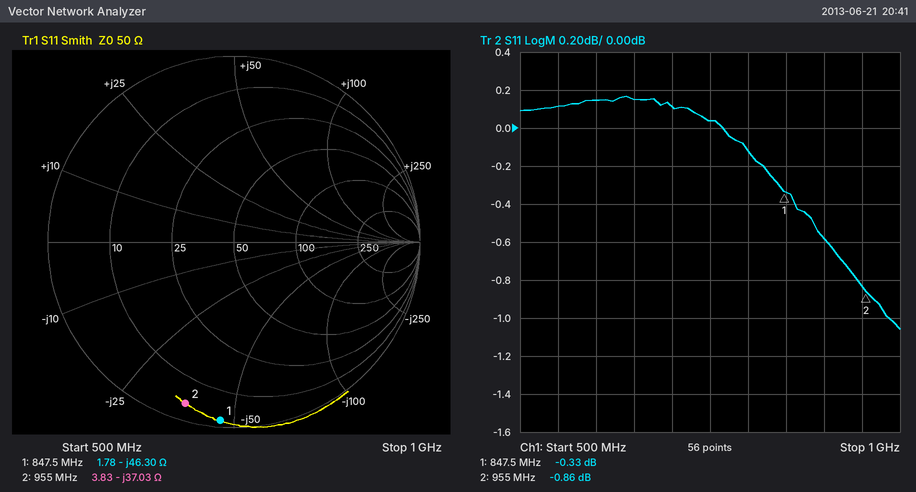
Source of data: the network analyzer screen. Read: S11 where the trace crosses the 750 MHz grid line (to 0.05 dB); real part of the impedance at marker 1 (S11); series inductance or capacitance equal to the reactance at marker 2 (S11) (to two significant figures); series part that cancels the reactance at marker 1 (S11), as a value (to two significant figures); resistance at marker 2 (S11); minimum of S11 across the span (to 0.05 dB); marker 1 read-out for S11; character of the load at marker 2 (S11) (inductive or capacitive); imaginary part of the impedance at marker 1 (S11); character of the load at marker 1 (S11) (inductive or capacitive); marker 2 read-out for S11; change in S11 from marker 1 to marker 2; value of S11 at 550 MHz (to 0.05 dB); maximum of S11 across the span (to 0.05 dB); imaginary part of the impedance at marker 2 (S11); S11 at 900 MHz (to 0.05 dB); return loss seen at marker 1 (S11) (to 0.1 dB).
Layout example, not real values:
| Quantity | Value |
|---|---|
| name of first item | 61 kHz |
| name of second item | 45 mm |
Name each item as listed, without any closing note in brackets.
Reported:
| Quantity | Value |
|---|---|
| S11 where the trace crosses the 750 MHz grid line | 0.05 dB |
| real part of the impedance at marker 1 | 1.78 Ω |
| series inductance or capacitance equal to the reactance at marker 2 (S11) | 4.5 pF |
| series part that cancels the reactance at marker 1 (S11), as a value | 8.7 nH |
| resistance at marker 2 | 3.83 Ω |
| minimum of S11 across the span | -1.05 dB |
| marker 1 read-out for S11 | -0.33 dB |
| character of the load at marker 2 (S11) | capacitive |
| imaginary part of the impedance at marker 1 | -46.30 Ω |
| character of the load at marker 1 (S11) | capacitive |
| marker 2 read-out for S11 | -0.86 dB |
| change in S11 from marker 1 to marker 2 | -0.53 dB |
| value of S11 at 550 MHz | 0.10 dB |
| maximum of S11 across the span | 0.15 dB |
| imaginary part of the impedance at marker 2 | -37.03 Ω |
| S11 at 900 MHz | -0.60 dB |
| return loss seen at marker 1 (S11) | 0.3 dB |
